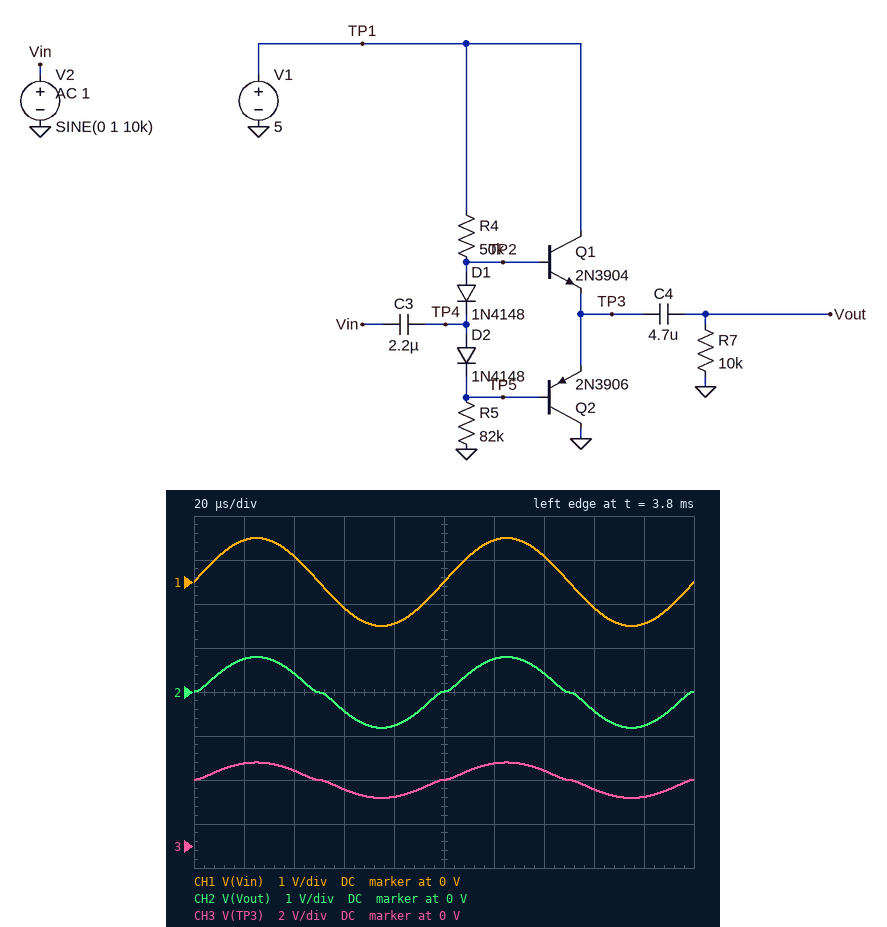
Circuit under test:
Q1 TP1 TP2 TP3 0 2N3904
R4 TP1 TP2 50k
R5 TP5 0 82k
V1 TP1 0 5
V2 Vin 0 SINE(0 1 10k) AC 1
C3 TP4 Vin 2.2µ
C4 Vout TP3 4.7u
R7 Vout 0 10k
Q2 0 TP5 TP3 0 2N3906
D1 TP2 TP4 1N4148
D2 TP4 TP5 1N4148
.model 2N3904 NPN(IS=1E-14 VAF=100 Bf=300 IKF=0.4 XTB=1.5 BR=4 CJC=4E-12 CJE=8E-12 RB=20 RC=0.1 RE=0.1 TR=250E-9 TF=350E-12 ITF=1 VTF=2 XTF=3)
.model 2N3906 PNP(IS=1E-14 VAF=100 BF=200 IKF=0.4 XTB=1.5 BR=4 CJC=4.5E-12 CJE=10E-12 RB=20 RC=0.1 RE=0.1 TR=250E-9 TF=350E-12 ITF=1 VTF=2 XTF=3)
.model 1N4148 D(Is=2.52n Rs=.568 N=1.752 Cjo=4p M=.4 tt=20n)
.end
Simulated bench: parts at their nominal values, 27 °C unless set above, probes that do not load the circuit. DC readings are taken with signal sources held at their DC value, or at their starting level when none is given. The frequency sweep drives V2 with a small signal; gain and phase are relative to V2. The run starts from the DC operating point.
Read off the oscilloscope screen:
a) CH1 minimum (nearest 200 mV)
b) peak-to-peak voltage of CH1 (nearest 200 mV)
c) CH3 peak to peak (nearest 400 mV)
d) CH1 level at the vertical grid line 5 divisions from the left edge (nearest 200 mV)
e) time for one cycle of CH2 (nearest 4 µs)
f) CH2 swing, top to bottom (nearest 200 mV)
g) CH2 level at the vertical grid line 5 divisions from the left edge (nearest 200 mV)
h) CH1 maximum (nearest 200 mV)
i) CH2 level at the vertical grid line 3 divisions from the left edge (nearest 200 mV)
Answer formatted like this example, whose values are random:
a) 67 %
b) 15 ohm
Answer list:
a) -1.0 V
b) 2.0 V
c) 1.6 V
d) 0 V
e) 100 µs
f) 1.6 V
g) 0 V
h) 1.0 V
i) -400 mV
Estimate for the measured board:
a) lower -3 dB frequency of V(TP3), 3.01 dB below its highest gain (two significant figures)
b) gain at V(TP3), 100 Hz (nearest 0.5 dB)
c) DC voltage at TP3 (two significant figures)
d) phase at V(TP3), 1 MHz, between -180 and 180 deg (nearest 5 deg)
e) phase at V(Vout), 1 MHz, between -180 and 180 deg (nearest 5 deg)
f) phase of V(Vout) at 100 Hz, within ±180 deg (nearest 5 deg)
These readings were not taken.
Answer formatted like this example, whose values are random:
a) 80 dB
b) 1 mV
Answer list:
a) 650 kHz
b) -19.5 dB
c) 3.0 V
d) 30 deg
e) 30 deg
f) 0 deg
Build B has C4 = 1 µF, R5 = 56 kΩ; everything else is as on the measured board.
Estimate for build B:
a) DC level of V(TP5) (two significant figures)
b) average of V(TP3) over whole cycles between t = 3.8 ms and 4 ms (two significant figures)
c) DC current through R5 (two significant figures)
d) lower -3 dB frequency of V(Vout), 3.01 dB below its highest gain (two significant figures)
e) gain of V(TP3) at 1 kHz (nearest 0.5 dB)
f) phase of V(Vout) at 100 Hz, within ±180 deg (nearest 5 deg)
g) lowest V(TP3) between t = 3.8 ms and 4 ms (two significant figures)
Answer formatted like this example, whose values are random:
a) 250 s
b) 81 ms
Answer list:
a) 2.2 V
b) 2.6 V
c) 39 µA
d) 680 kHz
e) -17.0 dB
f) 5 deg
g) 1.8 V
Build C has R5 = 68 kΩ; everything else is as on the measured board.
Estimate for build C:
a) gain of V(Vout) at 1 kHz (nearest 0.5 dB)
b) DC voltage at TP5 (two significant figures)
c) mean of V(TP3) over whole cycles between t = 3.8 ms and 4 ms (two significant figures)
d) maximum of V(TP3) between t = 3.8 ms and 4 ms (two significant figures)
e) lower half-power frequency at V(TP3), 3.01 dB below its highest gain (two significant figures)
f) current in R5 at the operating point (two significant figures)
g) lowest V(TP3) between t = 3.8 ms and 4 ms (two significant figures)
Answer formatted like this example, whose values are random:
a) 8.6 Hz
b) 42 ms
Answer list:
a) -18.0 dB
b) 2.4 V
c) 2.8 V
d) 3.6 V
e) 670 kHz
f) 35 µA
g) 2.0 V
